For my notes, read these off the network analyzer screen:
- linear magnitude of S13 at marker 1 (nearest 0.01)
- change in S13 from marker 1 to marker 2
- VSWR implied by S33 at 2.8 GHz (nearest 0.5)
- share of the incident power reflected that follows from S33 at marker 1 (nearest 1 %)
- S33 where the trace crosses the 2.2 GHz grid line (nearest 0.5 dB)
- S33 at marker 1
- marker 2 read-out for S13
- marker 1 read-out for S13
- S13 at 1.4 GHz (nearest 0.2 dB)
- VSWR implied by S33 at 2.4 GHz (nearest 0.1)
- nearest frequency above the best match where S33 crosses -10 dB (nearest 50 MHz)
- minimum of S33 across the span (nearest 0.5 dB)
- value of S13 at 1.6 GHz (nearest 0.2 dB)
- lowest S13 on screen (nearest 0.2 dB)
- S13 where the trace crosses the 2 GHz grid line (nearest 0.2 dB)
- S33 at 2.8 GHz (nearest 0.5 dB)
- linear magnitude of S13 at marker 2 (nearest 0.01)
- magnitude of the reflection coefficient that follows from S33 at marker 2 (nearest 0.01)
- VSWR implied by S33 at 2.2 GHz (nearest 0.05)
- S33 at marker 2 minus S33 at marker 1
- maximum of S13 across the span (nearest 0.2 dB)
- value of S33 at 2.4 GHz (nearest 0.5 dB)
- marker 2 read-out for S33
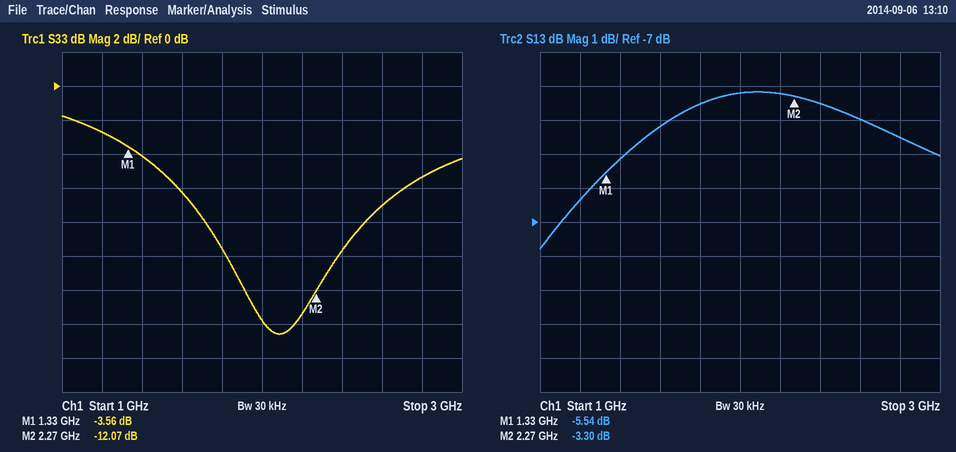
0.53
2.24 dB
3.5
44 %
-13.5 dB
-3.56 dB
-3.30 dB
-5.54 dB
-5.2 dB
2.0
2.40 GHz
-14.5 dB
-4.2 dB
-7.8 dB
-3.2 dB
-5.5 dB
0.68
0.25
1.55
-8.51 dB
-3.2 dB
-9.5 dB
-12.07 dB
